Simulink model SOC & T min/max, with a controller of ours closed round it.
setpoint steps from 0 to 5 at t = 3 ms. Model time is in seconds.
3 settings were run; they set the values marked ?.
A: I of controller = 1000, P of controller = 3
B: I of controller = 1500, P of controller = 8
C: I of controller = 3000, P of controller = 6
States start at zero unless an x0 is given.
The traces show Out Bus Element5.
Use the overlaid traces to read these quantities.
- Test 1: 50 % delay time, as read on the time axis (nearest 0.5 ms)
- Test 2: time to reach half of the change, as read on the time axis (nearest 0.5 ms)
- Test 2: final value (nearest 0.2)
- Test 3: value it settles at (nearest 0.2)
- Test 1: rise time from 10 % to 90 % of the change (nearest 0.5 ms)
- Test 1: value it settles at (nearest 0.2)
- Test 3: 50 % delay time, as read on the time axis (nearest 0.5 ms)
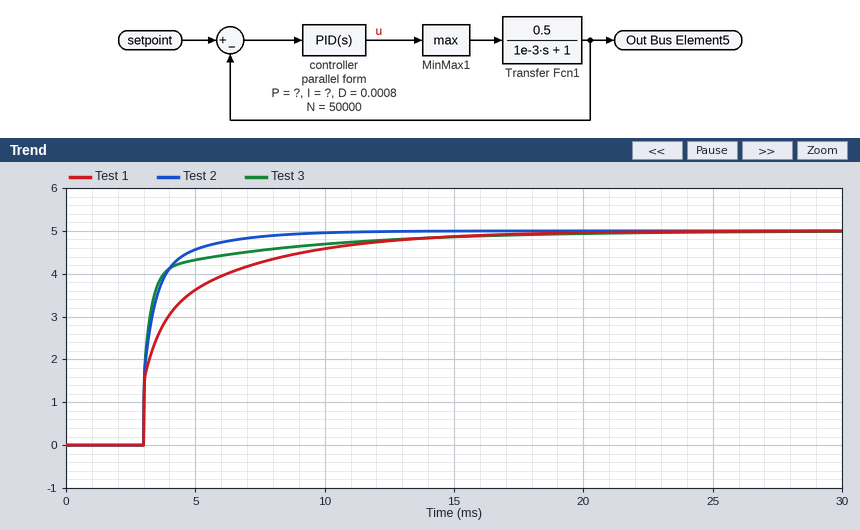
3.5 ms
3.0 ms
5.0
5.0
6.0 ms
5.0
3.0 ms
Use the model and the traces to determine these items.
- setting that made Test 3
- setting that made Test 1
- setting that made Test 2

B
A
C
